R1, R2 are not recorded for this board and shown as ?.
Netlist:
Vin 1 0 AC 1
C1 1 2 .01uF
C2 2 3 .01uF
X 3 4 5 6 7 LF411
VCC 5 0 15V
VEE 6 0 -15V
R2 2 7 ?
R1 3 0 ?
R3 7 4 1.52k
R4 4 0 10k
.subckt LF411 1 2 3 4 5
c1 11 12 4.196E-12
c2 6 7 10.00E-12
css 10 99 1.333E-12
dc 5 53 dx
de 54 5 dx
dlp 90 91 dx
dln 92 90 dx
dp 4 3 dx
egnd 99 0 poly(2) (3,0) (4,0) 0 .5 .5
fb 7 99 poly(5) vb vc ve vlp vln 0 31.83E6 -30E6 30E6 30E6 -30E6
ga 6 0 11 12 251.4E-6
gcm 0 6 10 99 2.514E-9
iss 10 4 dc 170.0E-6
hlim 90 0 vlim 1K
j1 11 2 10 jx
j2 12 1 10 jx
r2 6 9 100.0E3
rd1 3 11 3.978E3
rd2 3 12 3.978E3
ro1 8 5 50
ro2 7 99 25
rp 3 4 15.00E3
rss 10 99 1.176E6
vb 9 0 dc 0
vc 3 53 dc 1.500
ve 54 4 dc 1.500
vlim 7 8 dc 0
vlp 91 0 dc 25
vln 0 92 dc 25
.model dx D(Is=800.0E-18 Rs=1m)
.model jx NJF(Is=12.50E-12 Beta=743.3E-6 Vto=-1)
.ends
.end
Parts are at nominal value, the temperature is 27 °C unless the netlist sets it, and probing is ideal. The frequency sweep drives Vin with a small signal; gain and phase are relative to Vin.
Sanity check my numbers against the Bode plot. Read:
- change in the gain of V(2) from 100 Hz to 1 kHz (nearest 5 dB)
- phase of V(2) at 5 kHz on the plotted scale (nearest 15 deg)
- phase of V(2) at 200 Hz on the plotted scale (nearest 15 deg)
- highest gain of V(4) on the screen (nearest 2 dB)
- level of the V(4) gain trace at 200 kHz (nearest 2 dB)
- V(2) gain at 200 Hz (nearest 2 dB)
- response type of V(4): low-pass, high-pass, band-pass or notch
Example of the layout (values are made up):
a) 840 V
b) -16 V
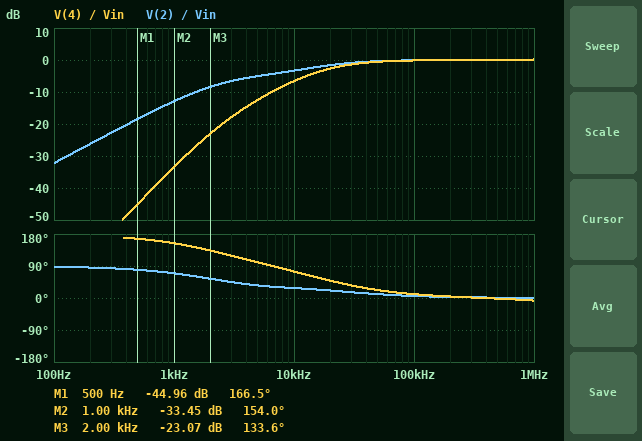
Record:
a) 20 dB
b) 30 deg
c) 90 deg
d) 0 dB
e) 0 dB
f) -26 dB
g) high-pass
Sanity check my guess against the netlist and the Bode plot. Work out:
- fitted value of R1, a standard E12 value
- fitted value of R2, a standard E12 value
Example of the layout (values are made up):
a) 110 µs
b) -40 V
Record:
a) 1.5 kΩ
b) 3.9 kΩ
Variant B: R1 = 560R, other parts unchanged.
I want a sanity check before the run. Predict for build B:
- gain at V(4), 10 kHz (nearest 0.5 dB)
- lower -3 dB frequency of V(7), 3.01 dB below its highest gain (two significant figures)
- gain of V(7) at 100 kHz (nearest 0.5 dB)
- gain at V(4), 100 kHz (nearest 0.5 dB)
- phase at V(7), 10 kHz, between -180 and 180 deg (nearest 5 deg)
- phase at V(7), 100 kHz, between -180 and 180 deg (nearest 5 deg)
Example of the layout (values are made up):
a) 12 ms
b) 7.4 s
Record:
a) -15.0 dB
b) 130 kHz
c) 0 dB
d) -1.0 dB
e) 90 deg
f) 30 deg
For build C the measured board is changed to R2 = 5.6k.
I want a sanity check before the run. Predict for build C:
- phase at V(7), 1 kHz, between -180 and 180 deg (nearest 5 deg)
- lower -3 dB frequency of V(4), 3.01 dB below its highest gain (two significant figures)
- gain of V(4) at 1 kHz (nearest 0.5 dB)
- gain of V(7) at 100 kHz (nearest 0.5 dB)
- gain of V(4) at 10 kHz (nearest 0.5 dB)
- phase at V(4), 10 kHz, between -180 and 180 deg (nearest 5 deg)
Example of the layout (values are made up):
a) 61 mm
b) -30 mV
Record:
a) 145 deg
b) 48 kHz
c) -31.0 dB
d) 1.0 dB
e) -7.0 dB
f) 70 deg
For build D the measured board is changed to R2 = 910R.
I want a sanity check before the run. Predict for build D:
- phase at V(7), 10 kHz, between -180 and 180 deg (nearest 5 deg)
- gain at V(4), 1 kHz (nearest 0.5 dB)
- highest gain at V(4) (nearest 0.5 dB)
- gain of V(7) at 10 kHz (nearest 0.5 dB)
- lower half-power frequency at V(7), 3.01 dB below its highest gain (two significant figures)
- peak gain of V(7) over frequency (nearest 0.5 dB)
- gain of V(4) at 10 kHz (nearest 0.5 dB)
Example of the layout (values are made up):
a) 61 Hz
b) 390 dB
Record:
a) 115 deg
b) -45.5 dB
c) 2.0 dB
d) -5.0 dB
e) 18 kHz
f) 3.0 dB
g) -6.0 dB
